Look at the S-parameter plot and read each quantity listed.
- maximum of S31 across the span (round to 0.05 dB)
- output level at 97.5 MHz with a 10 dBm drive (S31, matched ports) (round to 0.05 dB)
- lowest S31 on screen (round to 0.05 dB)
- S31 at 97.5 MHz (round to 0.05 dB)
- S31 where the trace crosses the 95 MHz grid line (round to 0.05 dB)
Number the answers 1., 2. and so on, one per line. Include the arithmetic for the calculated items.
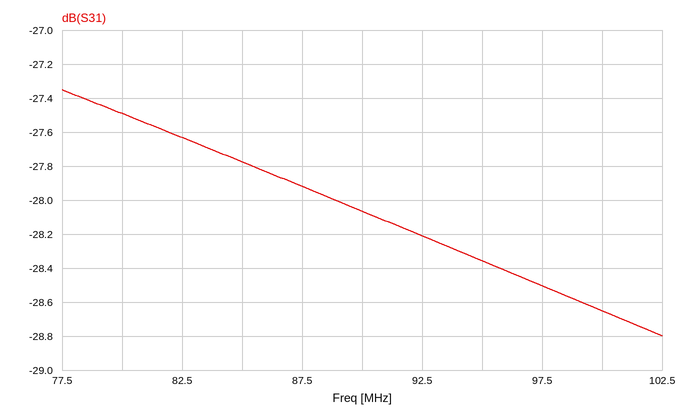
1. -27.35 dB
2. 10 dBm + (-28.50 dB) = -18.50 dBm
3. -28.80 dB
4. -28.50 dB
5. -28.35 dB
